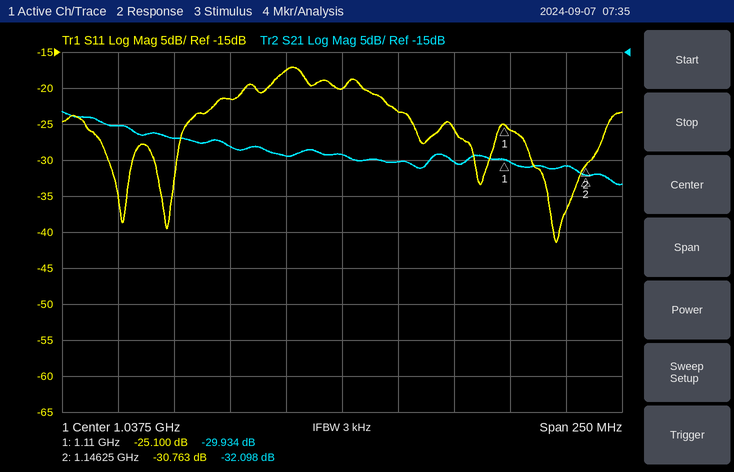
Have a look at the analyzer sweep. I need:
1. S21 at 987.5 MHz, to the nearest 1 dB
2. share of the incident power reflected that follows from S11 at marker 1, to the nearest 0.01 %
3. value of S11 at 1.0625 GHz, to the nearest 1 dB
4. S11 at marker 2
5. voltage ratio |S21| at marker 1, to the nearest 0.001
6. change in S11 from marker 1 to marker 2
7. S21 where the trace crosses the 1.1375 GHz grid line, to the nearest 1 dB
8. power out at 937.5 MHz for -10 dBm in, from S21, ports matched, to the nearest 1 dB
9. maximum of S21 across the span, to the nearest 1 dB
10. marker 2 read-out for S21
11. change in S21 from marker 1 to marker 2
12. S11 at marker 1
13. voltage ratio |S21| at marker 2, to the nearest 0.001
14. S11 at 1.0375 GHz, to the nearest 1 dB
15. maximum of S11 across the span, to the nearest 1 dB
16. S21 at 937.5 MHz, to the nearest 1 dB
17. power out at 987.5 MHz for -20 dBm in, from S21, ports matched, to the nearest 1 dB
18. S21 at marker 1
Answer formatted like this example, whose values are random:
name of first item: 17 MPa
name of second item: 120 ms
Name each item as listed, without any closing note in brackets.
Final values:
S21 at 987.5 MHz, to the nearest 1 dB: -28 dB
share of the incident power reflected that follows from S11 at marker 1, to the nearest 0.01 %: 0.31 %
value of S11 at 1.0625 GHz, to the nearest 1 dB: -23 dB
S11 at marker 2: -30.763 dB
voltage ratio |S21| at marker 1, to the nearest 0.001: 0.032
change in S11 from marker 1 to marker 2: -5.663 dB
S21 where the trace crosses the 1.1375 GHz grid line, to the nearest 1 dB: -31 dB
power out at 937.5 MHz for -10 dBm in, from S21, ports matched, to the nearest 1 dB: -35 dBm
maximum of S21 across the span, to the nearest 1 dB: -23 dB
marker 2 read-out for S21: -32.098 dB
change in S21 from marker 1 to marker 2: -2.164 dB
S11 at marker 1: -25.100 dB
voltage ratio |S21| at marker 2, to the nearest 0.001: 0.025
S11 at 1.0375 GHz, to the nearest 1 dB: -20 dB
maximum of S11 across the span, to the nearest 1 dB: -17 dB
S21 at 937.5 MHz, to the nearest 1 dB: -25 dB
power out at 987.5 MHz for -20 dBm in, from S21, ports matched, to the nearest 1 dB: -48 dBm
S21 at marker 1: -29.934 dB
